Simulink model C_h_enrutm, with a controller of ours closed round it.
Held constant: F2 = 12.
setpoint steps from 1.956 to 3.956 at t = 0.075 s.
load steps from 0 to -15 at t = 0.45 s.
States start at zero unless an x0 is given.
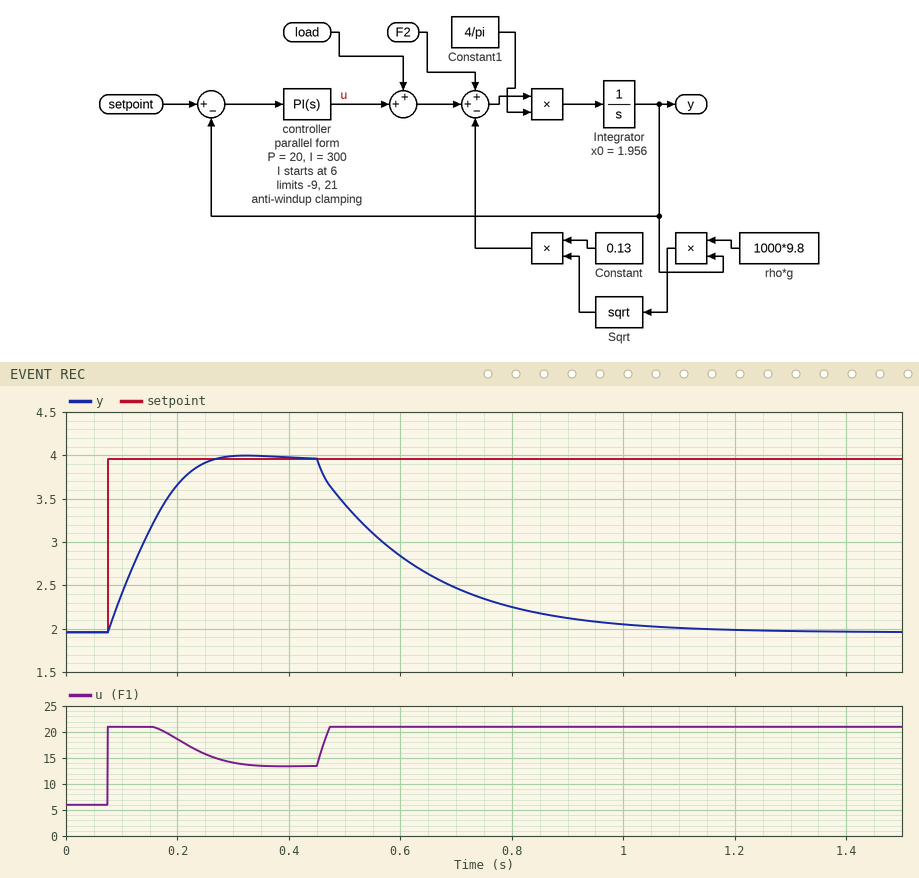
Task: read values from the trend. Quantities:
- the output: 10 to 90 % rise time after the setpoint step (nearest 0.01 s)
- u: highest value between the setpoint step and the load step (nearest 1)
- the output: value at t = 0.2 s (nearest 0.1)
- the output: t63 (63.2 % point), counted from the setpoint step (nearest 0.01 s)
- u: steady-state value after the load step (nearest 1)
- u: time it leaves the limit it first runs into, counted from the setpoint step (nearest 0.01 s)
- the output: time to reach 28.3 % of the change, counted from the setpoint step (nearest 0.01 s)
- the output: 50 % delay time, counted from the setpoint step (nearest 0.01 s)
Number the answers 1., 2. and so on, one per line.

1. 0.13 s
2. 21
3. 3.7
4. 0.08 s
5. 21
6. 0.09 s
7. 0.03 s
8. 0.06 s
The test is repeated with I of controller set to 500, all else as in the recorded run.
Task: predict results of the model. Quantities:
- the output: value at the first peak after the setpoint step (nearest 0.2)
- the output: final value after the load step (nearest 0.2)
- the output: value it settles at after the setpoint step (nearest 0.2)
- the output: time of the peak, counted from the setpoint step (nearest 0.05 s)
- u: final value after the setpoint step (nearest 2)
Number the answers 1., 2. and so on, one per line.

1. 4.0
2. 2.0
3. 4.0
4. 0.20 s
5. 14
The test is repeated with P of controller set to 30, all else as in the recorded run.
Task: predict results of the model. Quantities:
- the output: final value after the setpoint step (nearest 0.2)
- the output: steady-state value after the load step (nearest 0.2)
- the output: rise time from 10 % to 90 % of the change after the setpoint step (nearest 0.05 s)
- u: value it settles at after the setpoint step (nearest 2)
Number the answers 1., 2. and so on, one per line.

1. 4.0
2. 2.0
3. 0.15 s
4. 14
